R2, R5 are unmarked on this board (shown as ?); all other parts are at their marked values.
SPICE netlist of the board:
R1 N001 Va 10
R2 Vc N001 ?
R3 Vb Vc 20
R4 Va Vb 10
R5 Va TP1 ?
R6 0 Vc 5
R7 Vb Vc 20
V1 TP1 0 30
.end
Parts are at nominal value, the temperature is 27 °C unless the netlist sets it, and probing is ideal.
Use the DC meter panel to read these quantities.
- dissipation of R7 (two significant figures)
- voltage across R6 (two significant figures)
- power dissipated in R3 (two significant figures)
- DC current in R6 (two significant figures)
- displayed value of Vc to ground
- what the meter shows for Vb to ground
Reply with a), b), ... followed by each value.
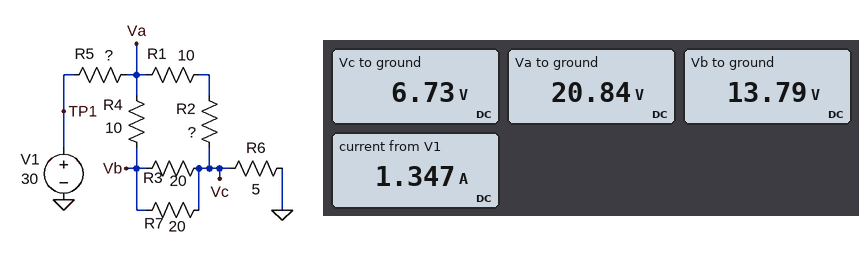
a) 2.5 W
b) 6.7 V
c) 2.5 W
d) 1.3 A
e) 6.73 V
f) 13.79 V
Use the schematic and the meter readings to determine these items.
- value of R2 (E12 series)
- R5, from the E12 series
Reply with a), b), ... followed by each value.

a) 12 Ω
b) 6.8 Ω
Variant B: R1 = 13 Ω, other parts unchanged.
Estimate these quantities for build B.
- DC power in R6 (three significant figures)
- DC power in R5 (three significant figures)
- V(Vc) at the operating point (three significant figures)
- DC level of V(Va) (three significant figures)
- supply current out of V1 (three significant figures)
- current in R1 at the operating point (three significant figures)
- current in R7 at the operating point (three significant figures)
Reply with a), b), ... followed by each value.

a) 8.57 W
b) 11.7 W
c) 6.55 V
d) 21.1 V
e) 1.31 A
f) 582 mA
g) 364 mA
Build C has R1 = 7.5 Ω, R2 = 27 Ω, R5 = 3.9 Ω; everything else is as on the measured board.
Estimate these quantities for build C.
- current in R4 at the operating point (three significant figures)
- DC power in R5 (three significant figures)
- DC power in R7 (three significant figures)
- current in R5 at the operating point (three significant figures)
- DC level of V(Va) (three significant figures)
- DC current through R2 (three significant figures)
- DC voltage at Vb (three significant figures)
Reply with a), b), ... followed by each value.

a) 881 mA
b) 7.55 W
c) 3.88 W
d) 1.39 A
e) 24.6 V
f) 511 mA
g) 15.8 V
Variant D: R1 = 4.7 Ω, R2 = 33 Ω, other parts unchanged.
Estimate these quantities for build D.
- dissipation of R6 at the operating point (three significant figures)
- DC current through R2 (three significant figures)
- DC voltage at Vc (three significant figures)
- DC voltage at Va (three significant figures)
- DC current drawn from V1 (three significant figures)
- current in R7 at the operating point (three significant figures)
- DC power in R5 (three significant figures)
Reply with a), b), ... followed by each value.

a) 7.28 W
b) 418 mA
c) 6.03 V
d) 21.8 V
e) 1.21 A
f) 394 mA
g) 9.90 W
